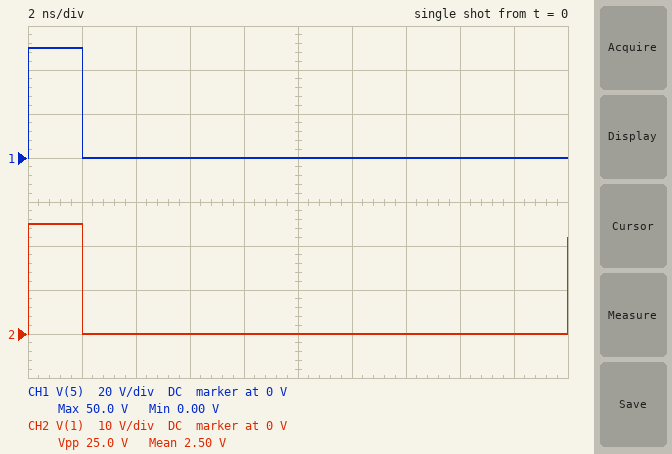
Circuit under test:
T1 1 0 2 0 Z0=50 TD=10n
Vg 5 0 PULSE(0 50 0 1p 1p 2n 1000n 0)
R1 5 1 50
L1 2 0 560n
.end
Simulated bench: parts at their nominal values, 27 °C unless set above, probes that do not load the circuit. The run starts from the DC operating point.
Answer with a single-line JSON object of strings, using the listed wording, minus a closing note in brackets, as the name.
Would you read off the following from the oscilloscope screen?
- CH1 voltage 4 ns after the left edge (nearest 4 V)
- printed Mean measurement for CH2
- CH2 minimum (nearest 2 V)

{"CH1 voltage 4 ns after the left edge": "0 V", "printed Mean measurement for CH2": "2.50 V", "CH2 minimum": "0 V"}
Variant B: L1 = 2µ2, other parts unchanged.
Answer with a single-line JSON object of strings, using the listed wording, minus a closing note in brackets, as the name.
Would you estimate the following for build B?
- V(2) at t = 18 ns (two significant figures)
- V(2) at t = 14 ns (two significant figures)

{"V(2) at t = 18 ns": "-1.9 V", "V(2) at t = 14 ns": "-2.1 V"}
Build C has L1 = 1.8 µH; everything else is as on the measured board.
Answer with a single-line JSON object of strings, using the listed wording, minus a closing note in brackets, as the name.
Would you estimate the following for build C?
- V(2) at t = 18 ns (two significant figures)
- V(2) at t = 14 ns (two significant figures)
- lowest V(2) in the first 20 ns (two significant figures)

{"V(2) at t = 18 ns": "-2.3 V", "V(2) at t = 14 ns": "-2.6 V", "lowest V(2) in the first 20 ns": "-2.7 V"}
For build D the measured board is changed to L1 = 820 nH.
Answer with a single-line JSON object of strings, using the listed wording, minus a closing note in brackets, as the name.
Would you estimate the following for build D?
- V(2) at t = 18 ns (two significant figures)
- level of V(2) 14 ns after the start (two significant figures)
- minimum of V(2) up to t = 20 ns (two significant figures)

{"V(2) at t = 18 ns": "-4.0 V", "level of V(2) 14 ns after the start": "-5.1 V", "minimum of V(2) up to t = 20 ns": "-5.7 V"}
